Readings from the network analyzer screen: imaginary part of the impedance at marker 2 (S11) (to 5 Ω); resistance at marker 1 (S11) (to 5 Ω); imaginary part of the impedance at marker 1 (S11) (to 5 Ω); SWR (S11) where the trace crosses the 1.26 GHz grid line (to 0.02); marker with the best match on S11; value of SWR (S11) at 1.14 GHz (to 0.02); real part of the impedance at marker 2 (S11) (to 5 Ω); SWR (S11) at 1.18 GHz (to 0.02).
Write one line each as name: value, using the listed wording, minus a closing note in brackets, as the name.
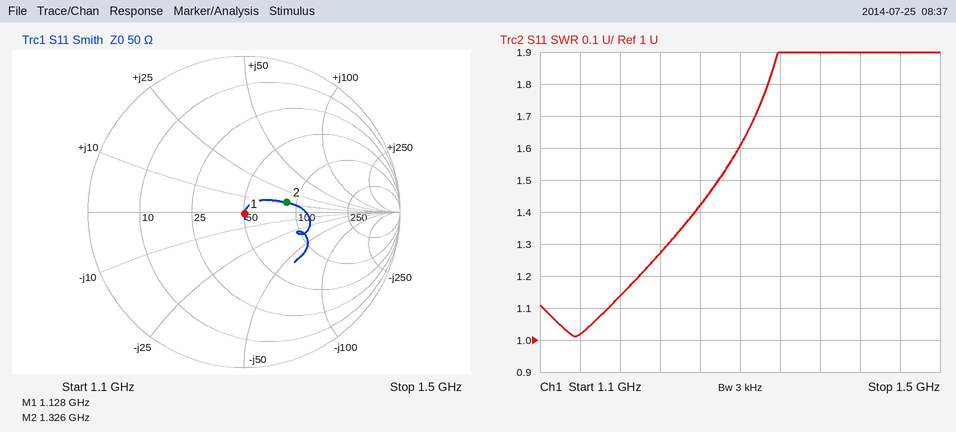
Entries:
imaginary part of the impedance at marker 2 (S11): +10 Ω
resistance at marker 1 (S11): 50 Ω
imaginary part of the impedance at marker 1 (S11): 0 Ω
SWR (S11) where the trace crosses the 1.26 GHz grid line: 1.42
marker with the best match on S11: marker 1
value of SWR (S11) at 1.14 GHz: 1.02
real part of the impedance at marker 2 (S11): 85 Ω
SWR (S11) at 1.18 GHz: 1.14
